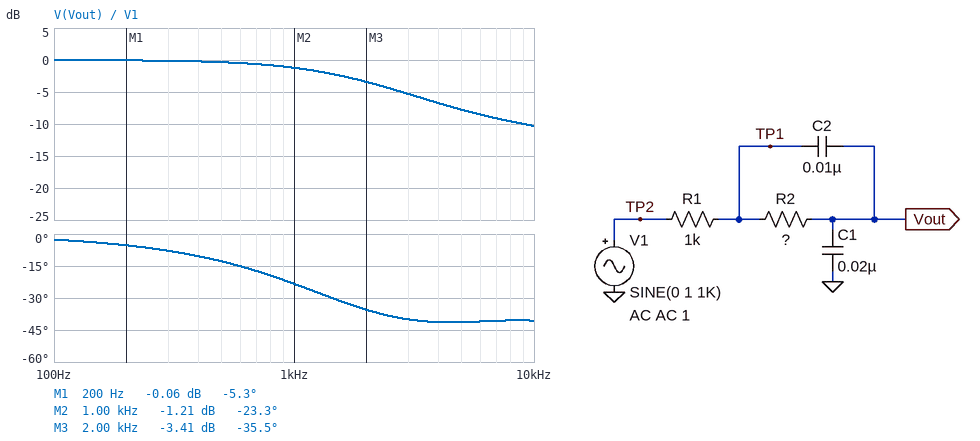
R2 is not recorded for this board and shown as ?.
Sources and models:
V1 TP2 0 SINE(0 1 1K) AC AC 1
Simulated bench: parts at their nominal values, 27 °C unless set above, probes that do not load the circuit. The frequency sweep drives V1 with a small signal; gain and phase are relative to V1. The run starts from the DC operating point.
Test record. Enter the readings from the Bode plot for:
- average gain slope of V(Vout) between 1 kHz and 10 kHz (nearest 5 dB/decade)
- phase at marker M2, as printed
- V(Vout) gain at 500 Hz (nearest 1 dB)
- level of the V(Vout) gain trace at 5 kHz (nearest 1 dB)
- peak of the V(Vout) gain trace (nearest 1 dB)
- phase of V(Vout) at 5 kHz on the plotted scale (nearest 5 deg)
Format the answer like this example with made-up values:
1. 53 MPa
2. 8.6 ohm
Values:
1. -10 dB/decade
2. -23.3 deg
3. 0 dB
4. -8 dB
5. 0 dB
6. -40 deg
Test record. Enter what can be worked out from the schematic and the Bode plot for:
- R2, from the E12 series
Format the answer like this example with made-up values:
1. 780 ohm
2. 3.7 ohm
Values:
1. 2.7 kΩ
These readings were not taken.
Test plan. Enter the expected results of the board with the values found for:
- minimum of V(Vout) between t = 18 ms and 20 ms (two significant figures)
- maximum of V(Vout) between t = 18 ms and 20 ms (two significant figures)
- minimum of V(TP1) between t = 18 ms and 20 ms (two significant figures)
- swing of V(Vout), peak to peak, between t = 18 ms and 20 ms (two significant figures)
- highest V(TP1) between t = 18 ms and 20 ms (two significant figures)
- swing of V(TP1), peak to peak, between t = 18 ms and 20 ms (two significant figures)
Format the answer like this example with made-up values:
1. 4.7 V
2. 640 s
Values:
1. -870 mV
2. 870 mV
3. -960 mV
4. 1.7 V
5. 960 mV
6. 1.9 V
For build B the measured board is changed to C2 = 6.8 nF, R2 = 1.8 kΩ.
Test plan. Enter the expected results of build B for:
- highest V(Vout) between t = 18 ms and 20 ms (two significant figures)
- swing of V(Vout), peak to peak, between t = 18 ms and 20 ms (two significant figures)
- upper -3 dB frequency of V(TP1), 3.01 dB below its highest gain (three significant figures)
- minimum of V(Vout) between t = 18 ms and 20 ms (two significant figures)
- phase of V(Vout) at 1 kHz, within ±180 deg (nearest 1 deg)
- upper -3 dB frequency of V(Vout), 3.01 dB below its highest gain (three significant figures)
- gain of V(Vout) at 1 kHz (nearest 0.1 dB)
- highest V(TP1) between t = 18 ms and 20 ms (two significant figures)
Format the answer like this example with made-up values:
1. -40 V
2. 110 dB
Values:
1. 930 mV
2. 1.9 V
3. 15.8 kHz
4. -930 mV
5. -19 deg
6. 2.55 kHz
7. -0.6 dB
8. 970 mV
